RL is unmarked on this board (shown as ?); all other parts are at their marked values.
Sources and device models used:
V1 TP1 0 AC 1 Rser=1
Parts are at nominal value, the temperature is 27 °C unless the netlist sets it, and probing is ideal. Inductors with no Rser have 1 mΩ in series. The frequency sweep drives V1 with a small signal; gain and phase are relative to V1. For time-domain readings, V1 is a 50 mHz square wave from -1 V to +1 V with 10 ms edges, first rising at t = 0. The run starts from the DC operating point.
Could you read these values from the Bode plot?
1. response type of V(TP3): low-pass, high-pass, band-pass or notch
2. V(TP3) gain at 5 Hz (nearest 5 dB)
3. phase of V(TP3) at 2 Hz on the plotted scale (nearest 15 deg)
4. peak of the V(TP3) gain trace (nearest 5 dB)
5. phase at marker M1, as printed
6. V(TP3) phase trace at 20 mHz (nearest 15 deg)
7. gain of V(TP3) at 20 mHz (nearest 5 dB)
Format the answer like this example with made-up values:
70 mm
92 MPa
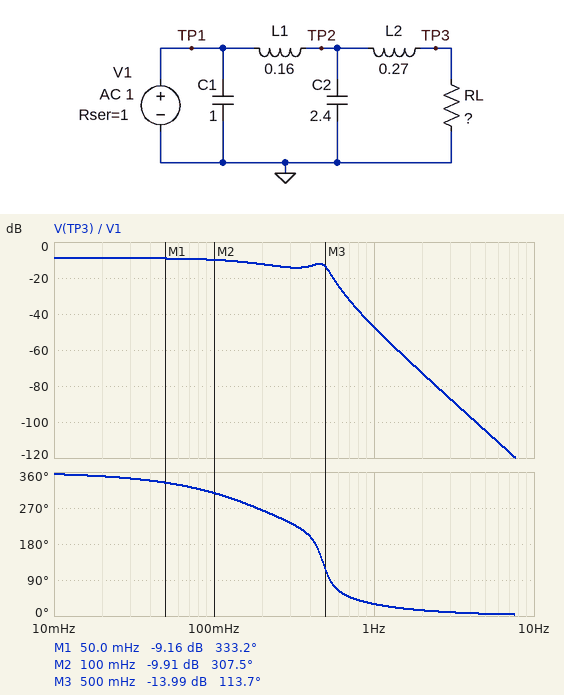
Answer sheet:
low-pass
-105 dB
15 deg
-10 dB
333.2 deg
345 deg
-10 dB
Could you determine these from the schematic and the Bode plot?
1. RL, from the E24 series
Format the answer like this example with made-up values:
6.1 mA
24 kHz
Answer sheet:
0.56 Ω
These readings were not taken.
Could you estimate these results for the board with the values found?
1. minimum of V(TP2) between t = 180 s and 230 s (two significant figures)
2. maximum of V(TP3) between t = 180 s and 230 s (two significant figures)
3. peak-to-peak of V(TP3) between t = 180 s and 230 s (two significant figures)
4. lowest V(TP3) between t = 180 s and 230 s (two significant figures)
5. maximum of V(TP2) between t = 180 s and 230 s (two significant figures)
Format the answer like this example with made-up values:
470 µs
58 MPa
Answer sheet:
-410 mV
380 mV
760 mV
-380 mV
410 mV
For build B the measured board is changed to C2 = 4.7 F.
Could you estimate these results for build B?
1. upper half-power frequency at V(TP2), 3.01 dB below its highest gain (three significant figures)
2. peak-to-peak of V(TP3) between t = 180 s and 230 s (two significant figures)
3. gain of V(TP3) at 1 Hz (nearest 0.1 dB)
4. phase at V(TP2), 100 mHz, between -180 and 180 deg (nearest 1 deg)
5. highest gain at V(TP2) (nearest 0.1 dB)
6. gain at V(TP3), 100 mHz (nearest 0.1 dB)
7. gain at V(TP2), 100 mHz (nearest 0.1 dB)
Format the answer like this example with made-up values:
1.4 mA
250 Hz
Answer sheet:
105 mHz
710 mV
-53.6 dB
-54 deg
-8.9 dB
-12.1 dB
-11.7 dB
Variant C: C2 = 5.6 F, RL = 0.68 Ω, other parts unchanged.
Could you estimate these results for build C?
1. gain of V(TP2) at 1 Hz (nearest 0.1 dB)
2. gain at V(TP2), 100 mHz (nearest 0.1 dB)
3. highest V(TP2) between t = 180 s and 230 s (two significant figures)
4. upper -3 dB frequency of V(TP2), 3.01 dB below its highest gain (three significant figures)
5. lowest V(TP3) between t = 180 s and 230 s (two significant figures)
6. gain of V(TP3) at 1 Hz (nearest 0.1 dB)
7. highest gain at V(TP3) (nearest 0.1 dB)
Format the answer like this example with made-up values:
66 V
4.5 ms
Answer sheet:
-45.2 dB
-12.5 dB
390 mV
70.1 mHz
-390 mV
-53.8 dB
-7.9 dB
